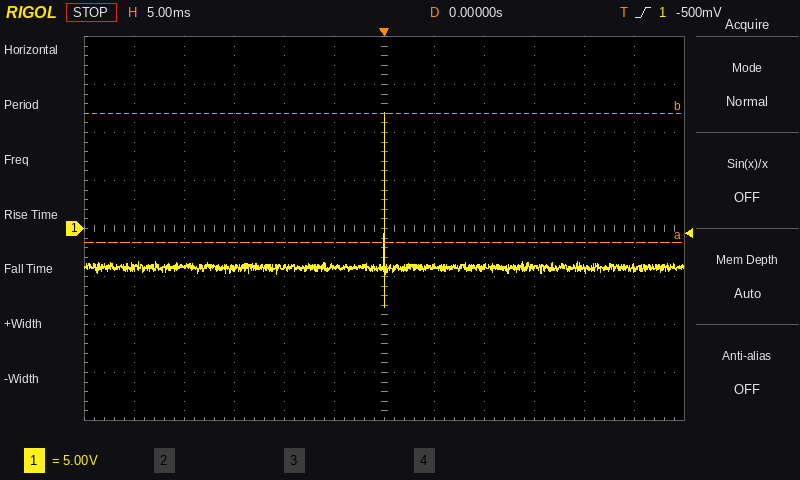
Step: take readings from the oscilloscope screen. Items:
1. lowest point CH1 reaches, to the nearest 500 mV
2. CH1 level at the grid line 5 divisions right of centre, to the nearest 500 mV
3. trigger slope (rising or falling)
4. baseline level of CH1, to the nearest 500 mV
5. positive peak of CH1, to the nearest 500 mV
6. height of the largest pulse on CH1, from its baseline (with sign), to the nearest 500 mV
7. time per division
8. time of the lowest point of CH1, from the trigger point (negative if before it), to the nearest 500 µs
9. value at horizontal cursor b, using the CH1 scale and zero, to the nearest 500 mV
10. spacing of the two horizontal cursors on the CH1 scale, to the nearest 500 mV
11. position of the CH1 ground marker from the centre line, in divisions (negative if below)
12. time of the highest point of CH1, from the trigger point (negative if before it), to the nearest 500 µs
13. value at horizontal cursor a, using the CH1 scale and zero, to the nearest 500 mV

-8.0 V
-4.0 V
rising
-4.0 V
12.0 V
+16.0 V
5 ms
0.0 ms
12.0 V
13.5 V
0.0 div
0.0 ms
-1.5 V
